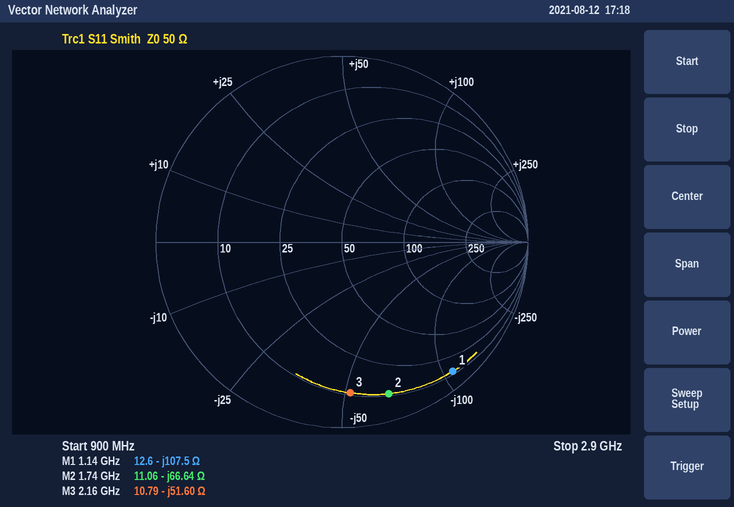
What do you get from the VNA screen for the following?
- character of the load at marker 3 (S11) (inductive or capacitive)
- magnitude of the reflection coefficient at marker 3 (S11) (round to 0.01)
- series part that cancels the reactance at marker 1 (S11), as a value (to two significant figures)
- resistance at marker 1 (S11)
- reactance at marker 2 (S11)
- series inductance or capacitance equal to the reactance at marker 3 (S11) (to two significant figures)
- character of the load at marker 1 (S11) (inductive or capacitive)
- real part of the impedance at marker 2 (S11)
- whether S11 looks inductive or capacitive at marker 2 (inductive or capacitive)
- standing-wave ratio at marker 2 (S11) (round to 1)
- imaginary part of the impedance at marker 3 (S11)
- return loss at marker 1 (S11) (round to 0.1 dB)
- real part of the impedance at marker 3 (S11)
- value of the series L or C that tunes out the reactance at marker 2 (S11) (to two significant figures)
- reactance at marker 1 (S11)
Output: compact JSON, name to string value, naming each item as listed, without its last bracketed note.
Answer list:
{"character of the load at marker 3 (S11)": "capacitive", "magnitude of the reflection coefficient at marker 3 (S11)": "0.81", "series part that cancels the reactance at marker 1 (S11), as a value": "15 nH", "resistance at marker 1": "12.6 Ω", "reactance at marker 2": "-66.64 Ω", "series inductance or capacitance equal to the reactance at marker 3 (S11)": "1.4 pF", "character of the load at marker 1 (S11)": "capacitive", "real part of the impedance at marker 2": "11.06 Ω", "whether S11 looks inductive or capacitive at marker 2": "capacitive", "standing-wave ratio at marker 2 (S11)": "13", "imaginary part of the impedance at marker 3": "-51.60 Ω", "return loss at marker 1 (S11)": "0.8 dB", "real part of the impedance at marker 3": "10.79 Ω", "value of the series L or C that tunes out the reactance at marker 2 (S11)": "6.1 nH", "reactance at marker 1": "-107.5 Ω"}
